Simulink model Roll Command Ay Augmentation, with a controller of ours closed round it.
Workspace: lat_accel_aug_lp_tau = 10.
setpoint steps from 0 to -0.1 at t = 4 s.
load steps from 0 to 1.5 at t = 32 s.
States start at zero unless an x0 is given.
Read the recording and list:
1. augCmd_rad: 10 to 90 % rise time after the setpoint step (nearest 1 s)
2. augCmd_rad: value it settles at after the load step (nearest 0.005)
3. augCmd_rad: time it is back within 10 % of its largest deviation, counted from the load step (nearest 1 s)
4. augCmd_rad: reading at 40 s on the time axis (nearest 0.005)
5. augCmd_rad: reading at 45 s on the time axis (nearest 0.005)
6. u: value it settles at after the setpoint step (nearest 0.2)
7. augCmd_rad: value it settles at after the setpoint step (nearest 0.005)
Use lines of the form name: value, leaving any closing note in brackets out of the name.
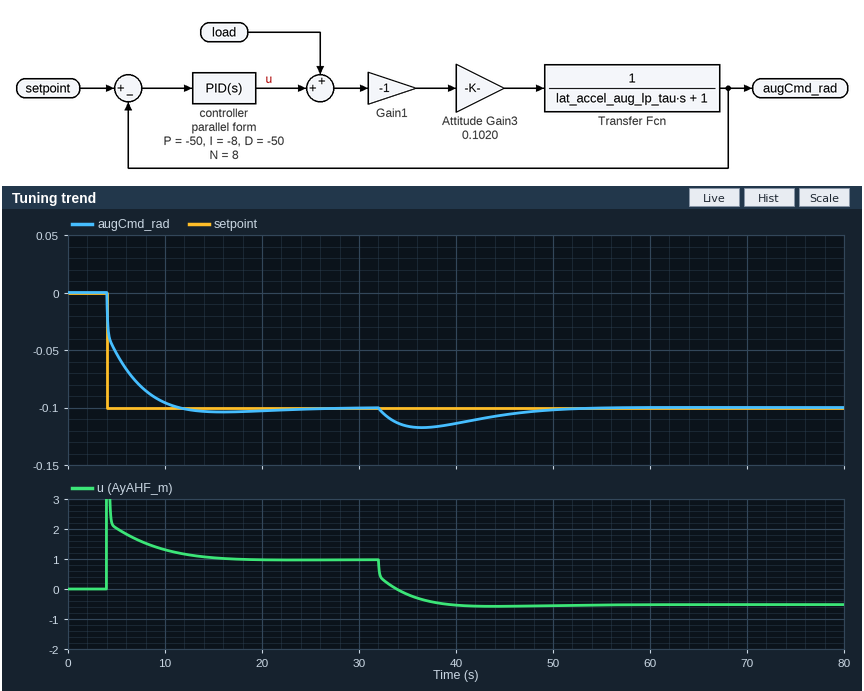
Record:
augCmd_rad: 10 to 90 % rise time after the setpoint step: 5 s
augCmd_rad: value it settles at after the load step: -0.100
augCmd_rad: time it is back within 10 % of its largest deviation, counted from the load step: 19 s
augCmd_rad: reading at 40 s on the time axis: -0.115
augCmd_rad: reading at 45 s on the time axis: -0.105
u: value it settles at after the setpoint step: 1.0
augCmd_rad: value it settles at after the setpoint step: -0.100
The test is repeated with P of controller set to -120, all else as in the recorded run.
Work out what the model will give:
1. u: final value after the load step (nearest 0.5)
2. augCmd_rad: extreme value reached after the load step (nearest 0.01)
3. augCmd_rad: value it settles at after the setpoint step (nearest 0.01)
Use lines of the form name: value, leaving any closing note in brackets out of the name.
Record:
u: final value after the load step: -0.5
augCmd_rad: extreme value reached after the load step: -0.11
augCmd_rad: value it settles at after the setpoint step: -0.10
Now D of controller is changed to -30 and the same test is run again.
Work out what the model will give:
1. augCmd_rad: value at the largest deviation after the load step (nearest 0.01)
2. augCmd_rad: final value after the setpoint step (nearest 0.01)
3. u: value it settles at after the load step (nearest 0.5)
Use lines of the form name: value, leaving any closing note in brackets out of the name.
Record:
augCmd_rad: value at the largest deviation after the load step: -0.12
augCmd_rad: final value after the setpoint step: -0.10
u: value it settles at after the load step: -0.5
